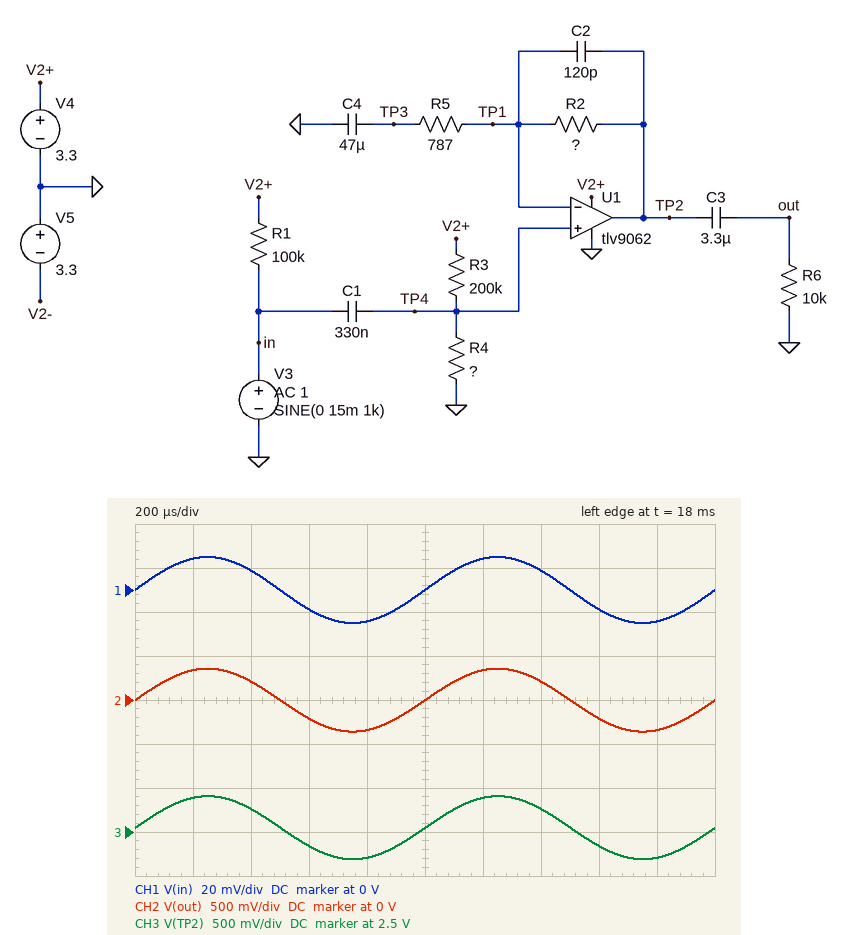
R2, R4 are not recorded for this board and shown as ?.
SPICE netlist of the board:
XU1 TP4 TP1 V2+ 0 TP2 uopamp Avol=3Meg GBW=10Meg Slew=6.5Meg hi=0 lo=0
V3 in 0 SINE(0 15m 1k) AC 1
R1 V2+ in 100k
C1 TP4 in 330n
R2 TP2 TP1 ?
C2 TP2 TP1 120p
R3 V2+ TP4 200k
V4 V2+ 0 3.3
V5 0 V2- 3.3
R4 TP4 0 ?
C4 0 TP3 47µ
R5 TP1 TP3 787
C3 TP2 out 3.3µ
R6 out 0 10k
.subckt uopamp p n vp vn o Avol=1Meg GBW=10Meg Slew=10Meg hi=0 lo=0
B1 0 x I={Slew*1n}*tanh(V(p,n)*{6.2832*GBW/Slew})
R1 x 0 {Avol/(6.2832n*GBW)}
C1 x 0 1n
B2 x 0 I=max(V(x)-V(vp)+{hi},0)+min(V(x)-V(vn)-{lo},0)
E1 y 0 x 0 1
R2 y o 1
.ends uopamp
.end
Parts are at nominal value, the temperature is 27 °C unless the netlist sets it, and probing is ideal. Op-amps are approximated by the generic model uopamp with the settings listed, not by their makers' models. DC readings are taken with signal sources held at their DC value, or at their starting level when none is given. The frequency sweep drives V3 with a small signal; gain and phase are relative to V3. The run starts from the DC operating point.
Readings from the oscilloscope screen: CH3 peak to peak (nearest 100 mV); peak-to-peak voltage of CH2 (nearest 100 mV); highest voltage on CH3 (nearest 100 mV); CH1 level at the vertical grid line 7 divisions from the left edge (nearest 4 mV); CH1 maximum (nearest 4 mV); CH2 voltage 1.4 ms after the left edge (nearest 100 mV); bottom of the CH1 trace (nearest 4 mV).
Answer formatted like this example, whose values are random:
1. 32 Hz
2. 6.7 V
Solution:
1. 700 mV
2. 700 mV
3. 2.9 V
4. 8 mV
5. 16 mV
6. 200 mV
7. -16 mV
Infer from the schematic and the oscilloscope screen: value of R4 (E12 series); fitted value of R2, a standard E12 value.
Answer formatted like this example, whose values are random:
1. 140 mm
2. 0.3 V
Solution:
1. 680 kΩ
2. 18 kΩ
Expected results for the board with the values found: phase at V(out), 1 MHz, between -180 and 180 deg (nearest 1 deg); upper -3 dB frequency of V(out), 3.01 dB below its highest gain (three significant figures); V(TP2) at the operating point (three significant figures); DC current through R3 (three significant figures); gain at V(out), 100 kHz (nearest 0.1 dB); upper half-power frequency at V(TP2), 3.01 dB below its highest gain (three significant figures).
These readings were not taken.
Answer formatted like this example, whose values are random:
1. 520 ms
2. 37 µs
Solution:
1. -62 deg
2. 63.1 kHz
3. 2.55 V
4. 3.75 µA
5. 22.1 dB
6. 63.1 kHz
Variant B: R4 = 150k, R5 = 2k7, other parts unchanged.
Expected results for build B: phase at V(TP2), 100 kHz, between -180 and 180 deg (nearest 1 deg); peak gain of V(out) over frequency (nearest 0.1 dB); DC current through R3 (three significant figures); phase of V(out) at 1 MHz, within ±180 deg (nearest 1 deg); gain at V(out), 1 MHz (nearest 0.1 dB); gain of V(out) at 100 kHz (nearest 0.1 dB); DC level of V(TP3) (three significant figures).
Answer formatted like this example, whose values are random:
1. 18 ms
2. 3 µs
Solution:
1. -45 deg
2. 17.7 dB
3. 9.43 µA
4. -31 deg
5. 0.7 dB
6. 13.0 dB
7. 1.41 V
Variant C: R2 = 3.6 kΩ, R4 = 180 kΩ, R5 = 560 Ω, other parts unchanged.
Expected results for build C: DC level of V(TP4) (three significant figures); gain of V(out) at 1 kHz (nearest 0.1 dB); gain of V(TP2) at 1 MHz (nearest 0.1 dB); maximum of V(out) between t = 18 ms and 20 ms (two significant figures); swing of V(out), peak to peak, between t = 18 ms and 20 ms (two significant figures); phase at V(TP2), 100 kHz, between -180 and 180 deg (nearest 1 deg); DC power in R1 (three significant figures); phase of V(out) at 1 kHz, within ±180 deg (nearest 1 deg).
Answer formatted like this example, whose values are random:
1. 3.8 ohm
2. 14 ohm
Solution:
1. 1.56 V
2. 17.4 dB
3. 7.0 dB
4. 110 mV
5. 220 mV
6. -17 deg
7. 109 µW
8. 1 deg
